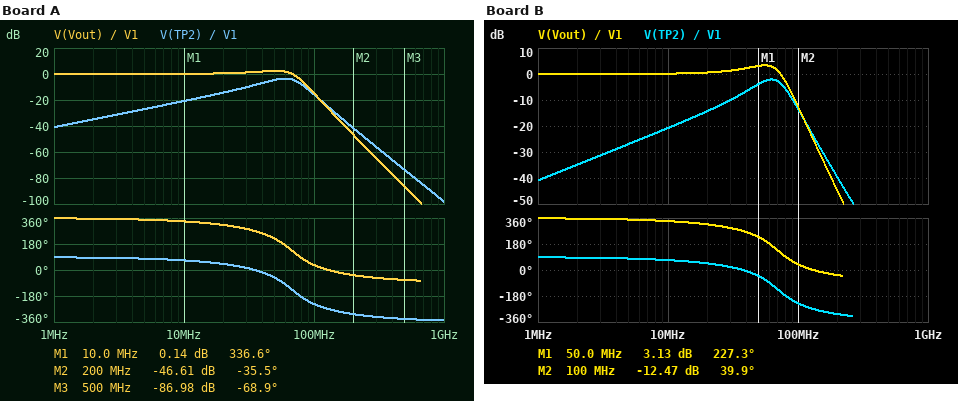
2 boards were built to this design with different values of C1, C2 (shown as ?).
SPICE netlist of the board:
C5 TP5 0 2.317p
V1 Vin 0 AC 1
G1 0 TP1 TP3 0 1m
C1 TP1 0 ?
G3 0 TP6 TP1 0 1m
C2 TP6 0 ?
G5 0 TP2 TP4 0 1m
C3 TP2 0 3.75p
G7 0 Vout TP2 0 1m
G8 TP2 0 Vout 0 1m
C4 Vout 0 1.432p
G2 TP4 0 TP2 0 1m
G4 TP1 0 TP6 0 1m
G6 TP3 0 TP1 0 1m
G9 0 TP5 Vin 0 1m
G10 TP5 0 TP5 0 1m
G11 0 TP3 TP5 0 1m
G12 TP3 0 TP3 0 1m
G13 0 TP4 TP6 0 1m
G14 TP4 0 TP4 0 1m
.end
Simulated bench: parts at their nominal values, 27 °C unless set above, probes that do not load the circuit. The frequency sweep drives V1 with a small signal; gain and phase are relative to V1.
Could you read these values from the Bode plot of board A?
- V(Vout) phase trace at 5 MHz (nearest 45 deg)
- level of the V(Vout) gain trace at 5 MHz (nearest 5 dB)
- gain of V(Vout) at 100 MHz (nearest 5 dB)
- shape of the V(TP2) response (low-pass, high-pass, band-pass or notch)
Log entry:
360 deg
0 dB
-15 dB
band-pass
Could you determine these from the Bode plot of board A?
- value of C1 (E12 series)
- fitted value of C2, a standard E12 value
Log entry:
2.2 pF
2.7 pF
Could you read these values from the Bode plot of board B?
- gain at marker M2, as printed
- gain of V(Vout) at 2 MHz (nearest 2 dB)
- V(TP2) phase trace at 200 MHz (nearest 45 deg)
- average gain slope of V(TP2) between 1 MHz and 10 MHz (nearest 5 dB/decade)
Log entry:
-12.47 dB
0 dB
-315 deg
20 dB/decade
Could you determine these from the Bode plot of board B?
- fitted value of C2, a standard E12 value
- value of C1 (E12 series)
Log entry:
2.2 pF
2.2 pF
